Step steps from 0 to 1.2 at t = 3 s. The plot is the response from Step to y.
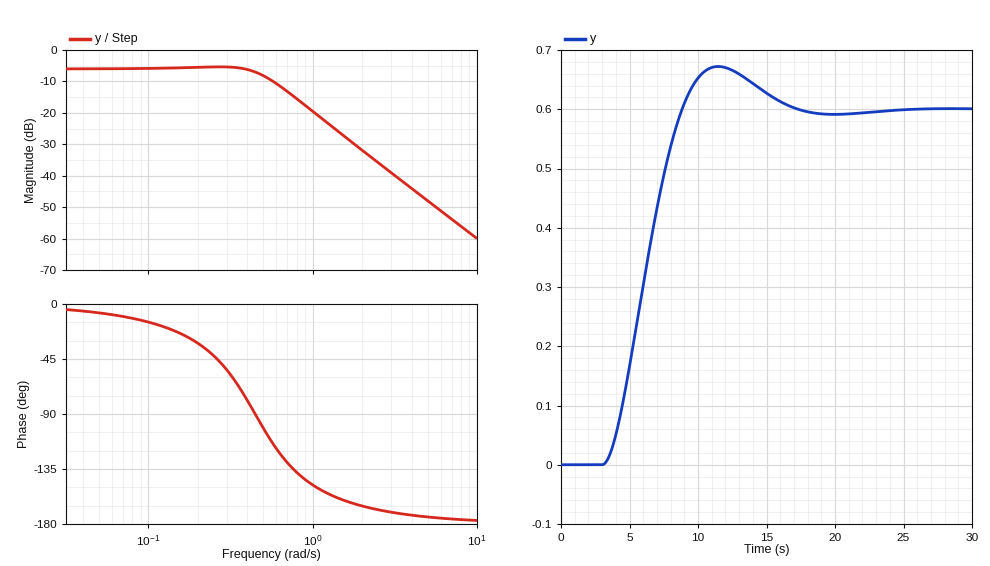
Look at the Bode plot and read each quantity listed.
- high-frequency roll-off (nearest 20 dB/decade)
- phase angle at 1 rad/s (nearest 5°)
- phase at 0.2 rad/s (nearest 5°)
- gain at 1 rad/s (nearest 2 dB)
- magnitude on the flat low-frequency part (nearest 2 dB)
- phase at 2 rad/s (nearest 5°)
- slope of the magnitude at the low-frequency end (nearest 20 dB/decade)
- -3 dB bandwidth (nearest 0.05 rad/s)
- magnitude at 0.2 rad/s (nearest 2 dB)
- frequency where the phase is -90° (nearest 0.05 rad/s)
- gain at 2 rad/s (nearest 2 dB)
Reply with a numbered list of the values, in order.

1. -40 dB/decade
2. -150°
3. -30°
4. -20 dB
5. -6 dB
6. -165°
7. 0 dB/decade
8. 0.55 rad/s
9. -6 dB
10. 0.45 rad/s
11. -32 dB
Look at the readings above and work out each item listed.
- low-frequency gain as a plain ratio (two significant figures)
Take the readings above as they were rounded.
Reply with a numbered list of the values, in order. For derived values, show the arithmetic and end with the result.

1. 10^(-6 / 20) = 0.50
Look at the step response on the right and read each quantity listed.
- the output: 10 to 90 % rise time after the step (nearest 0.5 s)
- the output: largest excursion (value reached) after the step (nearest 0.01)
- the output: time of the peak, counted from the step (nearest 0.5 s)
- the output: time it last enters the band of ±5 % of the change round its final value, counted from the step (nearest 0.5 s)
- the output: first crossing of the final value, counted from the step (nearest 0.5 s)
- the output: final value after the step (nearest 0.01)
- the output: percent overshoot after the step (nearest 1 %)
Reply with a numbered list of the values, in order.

1. 4.0 s
2. 0.67
3. 8.5 s
4. 12.0 s
5. 6.0 s
6. 0.60
7. 12 %
